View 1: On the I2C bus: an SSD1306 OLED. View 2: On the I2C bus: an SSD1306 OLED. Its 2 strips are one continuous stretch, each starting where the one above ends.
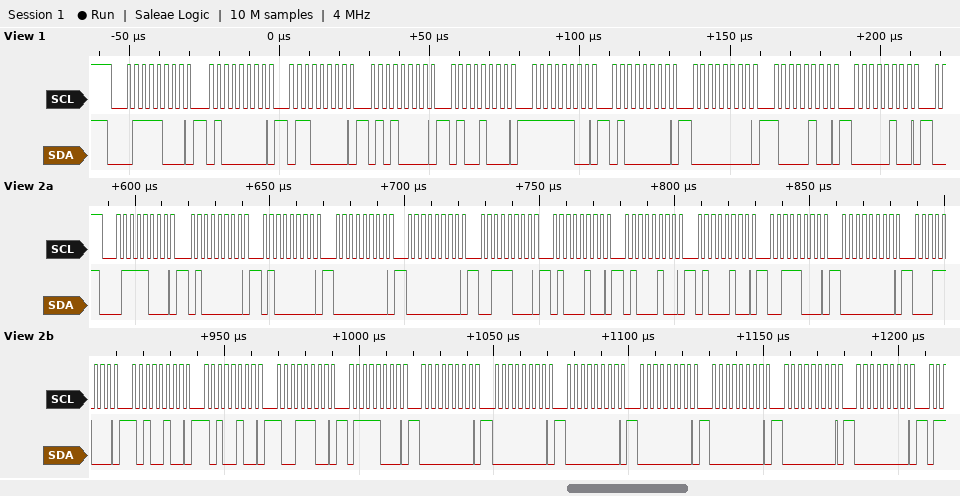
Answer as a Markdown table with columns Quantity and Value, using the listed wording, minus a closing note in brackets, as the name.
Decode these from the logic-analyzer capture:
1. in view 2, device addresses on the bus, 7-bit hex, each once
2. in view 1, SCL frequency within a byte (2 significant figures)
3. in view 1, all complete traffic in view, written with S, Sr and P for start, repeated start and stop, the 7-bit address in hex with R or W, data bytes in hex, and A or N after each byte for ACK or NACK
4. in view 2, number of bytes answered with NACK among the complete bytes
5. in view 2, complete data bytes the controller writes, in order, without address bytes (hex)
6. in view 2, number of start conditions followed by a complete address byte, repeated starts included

| Quantity | Value |
|---|---|
| in view 2, device addresses on the bus, 7-bit hex, each once | 0x3C |
| in view 1, SCL frequency within a byte | 400 kHz |
| in view 1, all complete traffic in view, written with S, Sr and P for start, repeated start and stop, the 7-bit address in hex with R or W, data bytes in hex, and A or N after each byte for ACK or NACK | S 3CW A 40 A 60 A 50 A 48 A FC A 40 A 00 A 84 A 04 A |
| in view 2, number of bytes answered with NACK among the complete bytes | 0 |
| in view 2, complete data bytes the controller writes, in order, without address bytes | 40 40 00 00 38 44 44 44 38 00 18 A4 A4 9C 78 00 00 00 00 00 00 00 |
| in view 2, number of start conditions followed by a complete address byte, repeated starts included | 1 |
